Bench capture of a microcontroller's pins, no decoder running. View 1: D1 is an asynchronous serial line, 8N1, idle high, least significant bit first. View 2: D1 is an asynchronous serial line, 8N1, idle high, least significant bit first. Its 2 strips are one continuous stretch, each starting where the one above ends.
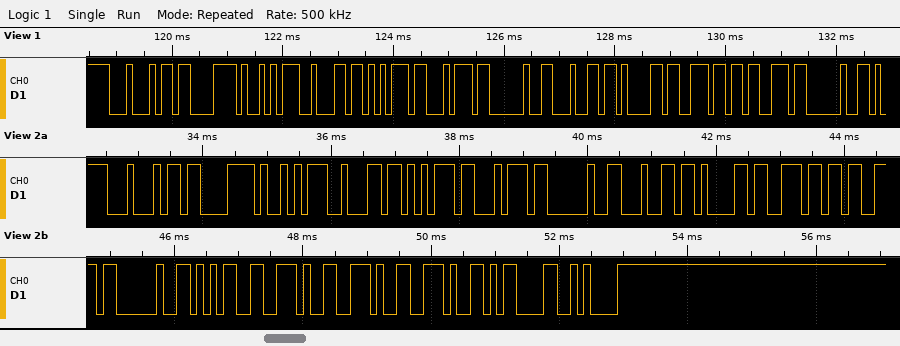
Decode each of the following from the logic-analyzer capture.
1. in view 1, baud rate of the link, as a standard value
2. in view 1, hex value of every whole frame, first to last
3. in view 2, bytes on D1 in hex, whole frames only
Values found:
9600 baud
44 C3 A9 62 75 74 20 64 61 6E 73 20
44 C3 A9 62 75 74 20 64 61 6E 73 20 35 2E 2E 2E 0D 0A
